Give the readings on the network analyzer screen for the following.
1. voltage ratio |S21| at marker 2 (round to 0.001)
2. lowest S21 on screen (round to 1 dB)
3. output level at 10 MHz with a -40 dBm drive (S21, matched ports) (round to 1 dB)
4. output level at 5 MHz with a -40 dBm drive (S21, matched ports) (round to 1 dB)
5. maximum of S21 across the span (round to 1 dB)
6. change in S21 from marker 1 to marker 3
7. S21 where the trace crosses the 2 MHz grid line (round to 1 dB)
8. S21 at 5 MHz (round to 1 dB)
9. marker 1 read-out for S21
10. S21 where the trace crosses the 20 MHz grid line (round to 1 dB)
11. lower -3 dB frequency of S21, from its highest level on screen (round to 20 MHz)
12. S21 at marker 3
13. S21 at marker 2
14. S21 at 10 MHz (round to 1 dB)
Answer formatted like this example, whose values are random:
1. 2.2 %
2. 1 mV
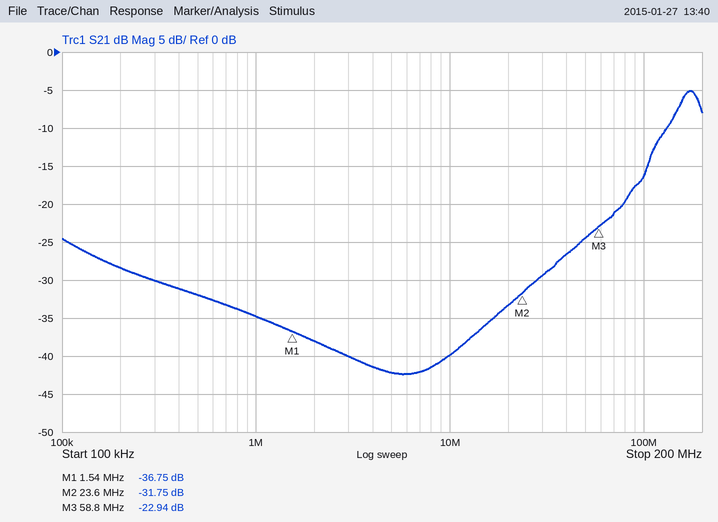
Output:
1. 0.026
2. -42 dB
3. -80 dBm
4. -82 dBm
5. -5 dB
6. 13.81 dB
7. -38 dB
8. -42 dB
9. -36.75 dB
10. -33 dB
11. 140 MHz
12. -22.94 dB
13. -31.75 dB
14. -40 dB
